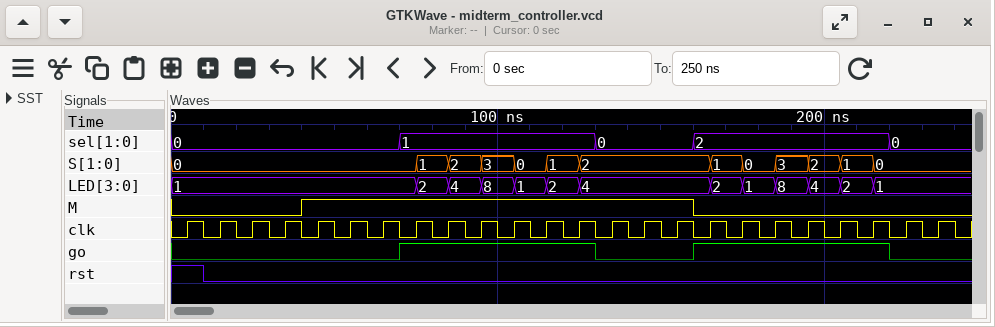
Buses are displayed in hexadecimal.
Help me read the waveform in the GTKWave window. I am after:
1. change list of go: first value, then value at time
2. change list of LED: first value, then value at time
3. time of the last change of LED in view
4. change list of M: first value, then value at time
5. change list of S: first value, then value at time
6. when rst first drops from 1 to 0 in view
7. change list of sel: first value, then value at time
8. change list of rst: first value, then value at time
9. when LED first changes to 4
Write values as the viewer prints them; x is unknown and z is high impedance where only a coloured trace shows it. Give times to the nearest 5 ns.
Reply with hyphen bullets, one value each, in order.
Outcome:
- 0, 1 at 70 ns, 0 at 130 ns, 1 at 160 ns, 0 at 220 ns
- 1, 2 at 75 ns, 4 at 85 ns, 8 at 95 ns, 1 at 105 ns, 2 at 115 ns, 4 at 125 ns, 2 at 165 ns, 1 at 175 ns, 8 at 185 ns, 4 at 195 ns, 2 at 205 ns, 1 at 215 ns
- 215 ns
- 0, 1 at 40 ns, 0 at 160 ns
- 0, 1 at 75 ns, 2 at 85 ns, 3 at 95 ns, 0 at 105 ns, 1 at 115 ns, 2 at 125 ns, 1 at 165 ns, 0 at 175 ns, 3 at 185 ns, 2 at 195 ns, 1 at 205 ns, 0 at 215 ns
- 10 ns
- 0, 1 at 70 ns, 0 at 130 ns, 2 at 160 ns, 0 at 220 ns
- 1, 0 at 10 ns
- 85 ns
